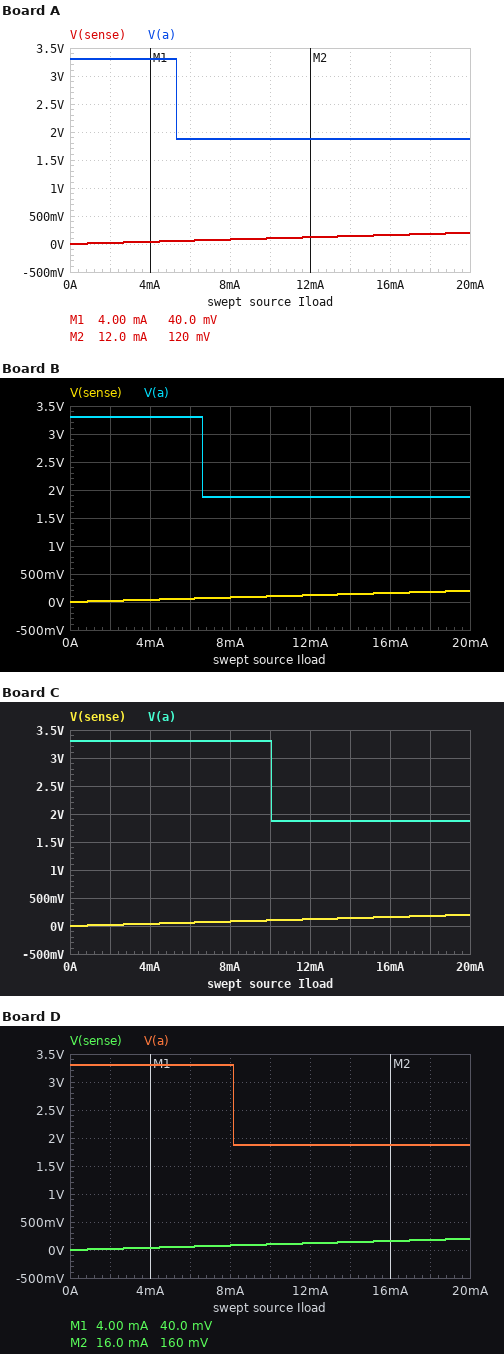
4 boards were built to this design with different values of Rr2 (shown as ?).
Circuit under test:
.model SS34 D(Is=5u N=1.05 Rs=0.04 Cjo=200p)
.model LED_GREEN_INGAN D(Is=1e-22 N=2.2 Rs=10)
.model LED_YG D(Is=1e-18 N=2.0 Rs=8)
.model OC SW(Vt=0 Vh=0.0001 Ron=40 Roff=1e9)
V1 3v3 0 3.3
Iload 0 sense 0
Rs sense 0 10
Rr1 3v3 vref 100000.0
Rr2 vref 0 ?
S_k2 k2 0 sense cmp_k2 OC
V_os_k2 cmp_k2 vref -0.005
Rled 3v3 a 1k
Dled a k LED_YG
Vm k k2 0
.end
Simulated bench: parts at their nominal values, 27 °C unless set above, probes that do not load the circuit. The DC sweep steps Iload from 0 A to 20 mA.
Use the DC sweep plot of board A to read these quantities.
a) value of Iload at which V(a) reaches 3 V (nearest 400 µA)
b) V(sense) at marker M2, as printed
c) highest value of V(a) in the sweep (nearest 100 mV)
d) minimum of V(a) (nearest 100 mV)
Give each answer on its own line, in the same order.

5.2 mA
120 mV
3.3 V
1.9 V
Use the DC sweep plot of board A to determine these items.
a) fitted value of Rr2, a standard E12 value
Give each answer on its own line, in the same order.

1.8 kΩ
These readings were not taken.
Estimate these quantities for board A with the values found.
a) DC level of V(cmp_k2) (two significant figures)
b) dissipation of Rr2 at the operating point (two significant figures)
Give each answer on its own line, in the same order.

53 mV
1.9 µW
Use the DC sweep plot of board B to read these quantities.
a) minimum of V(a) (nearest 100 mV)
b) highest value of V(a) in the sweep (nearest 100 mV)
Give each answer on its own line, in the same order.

1.9 V
3.3 V
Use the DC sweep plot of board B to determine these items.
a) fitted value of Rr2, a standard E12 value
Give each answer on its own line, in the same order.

2.2 kΩ
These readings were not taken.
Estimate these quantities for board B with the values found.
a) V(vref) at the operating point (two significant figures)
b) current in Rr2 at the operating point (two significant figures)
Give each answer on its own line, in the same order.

71 mV
32 µA
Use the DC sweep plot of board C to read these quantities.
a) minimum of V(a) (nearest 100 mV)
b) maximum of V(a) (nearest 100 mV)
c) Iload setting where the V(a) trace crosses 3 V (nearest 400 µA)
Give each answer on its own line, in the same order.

1.9 V
3.3 V
10.0 mA
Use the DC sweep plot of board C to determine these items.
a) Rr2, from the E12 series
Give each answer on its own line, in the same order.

3.3 kΩ
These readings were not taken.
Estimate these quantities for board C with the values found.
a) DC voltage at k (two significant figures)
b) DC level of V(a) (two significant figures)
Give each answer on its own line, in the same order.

2.2 V
3.3 V
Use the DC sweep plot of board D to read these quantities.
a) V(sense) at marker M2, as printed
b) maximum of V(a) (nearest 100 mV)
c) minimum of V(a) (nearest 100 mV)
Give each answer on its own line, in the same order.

160 mV
3.3 V
1.9 V
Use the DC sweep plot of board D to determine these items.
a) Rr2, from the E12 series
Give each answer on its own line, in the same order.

2.7 kΩ
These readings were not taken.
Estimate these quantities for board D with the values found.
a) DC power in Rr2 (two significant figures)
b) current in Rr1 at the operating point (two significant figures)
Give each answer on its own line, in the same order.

2.8 µW
32 µA
